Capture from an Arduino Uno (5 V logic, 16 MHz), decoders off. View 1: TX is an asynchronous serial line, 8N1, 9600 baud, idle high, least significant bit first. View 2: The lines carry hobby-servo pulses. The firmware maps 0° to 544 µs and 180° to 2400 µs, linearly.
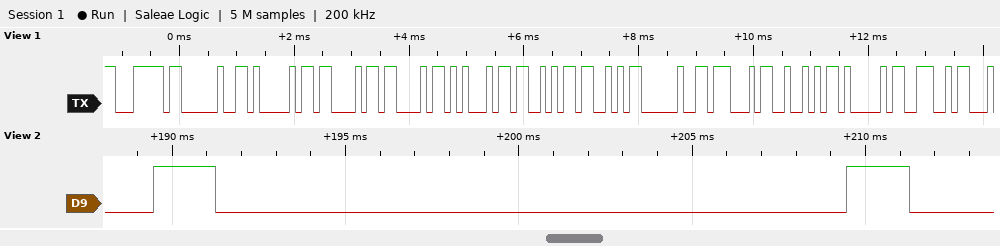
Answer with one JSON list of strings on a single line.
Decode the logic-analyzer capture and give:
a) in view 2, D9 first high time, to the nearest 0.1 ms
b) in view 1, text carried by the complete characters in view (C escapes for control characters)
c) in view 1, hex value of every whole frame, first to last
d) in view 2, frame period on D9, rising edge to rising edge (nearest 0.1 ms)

["1.8 ms", "\"| ACCESS GRAN\"", "7C 20 41 43 43 45 53 53 20 47 52 41 4E", "20.0 ms"]
